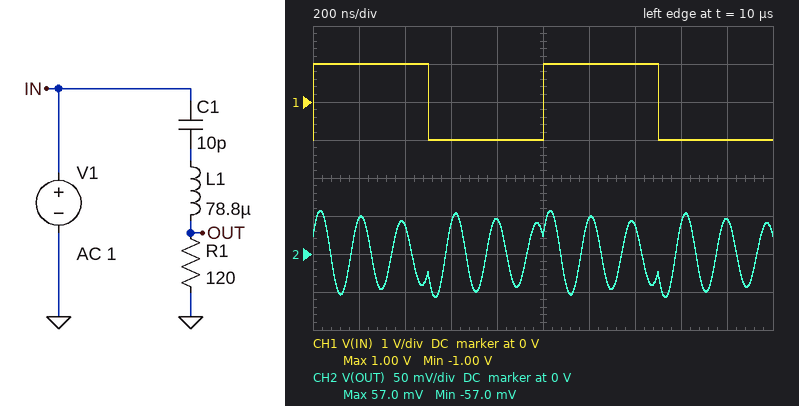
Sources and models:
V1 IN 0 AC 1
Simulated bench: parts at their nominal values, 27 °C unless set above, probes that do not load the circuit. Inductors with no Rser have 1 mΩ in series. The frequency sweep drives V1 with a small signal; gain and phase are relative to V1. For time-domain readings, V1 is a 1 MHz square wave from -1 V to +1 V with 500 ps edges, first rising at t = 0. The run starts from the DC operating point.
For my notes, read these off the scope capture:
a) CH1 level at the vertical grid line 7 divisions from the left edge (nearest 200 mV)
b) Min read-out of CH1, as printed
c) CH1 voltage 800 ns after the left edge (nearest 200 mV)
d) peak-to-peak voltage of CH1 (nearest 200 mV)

1.0 V
-1.00 V
-1.0 V
2.0 V
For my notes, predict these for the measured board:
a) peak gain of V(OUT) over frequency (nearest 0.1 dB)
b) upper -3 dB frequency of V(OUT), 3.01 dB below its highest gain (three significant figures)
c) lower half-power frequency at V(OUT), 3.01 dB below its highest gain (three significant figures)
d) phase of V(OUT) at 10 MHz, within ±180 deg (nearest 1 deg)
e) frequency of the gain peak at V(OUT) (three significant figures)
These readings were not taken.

0 dB
5.79 MHz
5.55 MHz
-88 deg
5.67 MHz
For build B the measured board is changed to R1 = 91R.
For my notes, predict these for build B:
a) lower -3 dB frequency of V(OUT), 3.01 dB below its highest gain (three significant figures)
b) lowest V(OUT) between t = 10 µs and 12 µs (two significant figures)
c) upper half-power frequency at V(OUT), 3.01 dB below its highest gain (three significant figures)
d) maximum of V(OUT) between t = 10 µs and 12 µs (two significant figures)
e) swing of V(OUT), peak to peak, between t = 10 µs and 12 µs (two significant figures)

5.58 MHz
-42 mV
5.76 MHz
42 mV
84 mV
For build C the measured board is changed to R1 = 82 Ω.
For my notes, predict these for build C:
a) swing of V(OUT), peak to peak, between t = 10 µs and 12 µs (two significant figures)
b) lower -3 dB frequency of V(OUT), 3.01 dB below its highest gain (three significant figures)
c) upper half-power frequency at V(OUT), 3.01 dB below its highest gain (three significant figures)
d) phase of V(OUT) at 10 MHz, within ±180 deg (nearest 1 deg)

75 mV
5.59 MHz
5.75 MHz
-89 deg
